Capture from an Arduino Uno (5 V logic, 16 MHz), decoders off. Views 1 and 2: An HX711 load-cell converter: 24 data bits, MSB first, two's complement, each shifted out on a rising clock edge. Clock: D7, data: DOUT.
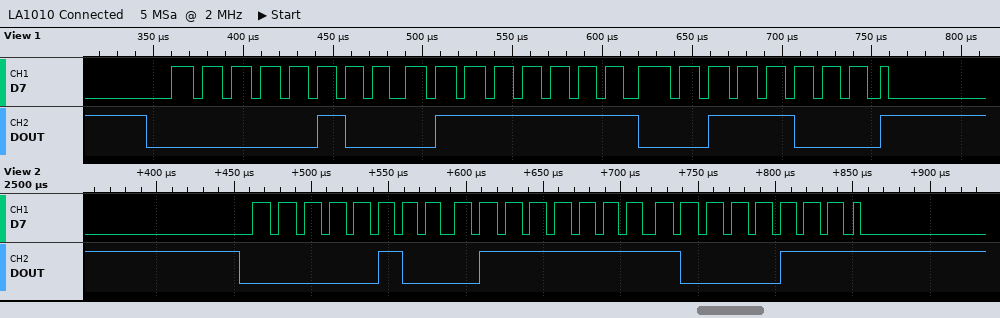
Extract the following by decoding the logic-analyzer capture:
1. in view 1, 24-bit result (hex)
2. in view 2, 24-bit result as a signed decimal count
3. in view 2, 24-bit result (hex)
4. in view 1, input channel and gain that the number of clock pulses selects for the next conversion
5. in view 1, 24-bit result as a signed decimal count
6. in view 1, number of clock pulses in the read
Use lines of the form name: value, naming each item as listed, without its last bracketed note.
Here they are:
in view 1, 24-bit result: 0x047F38
in view 2, 24-bit result as a signed decimal count: 294791
in view 2, 24-bit result: 0x047F87
in view 1, input channel and gain that the number of clock pulses selects for the next conversion: channel A, gain 128
in view 1, 24-bit result as a signed decimal count: 294712
in view 1, number of clock pulses in the read: 25
